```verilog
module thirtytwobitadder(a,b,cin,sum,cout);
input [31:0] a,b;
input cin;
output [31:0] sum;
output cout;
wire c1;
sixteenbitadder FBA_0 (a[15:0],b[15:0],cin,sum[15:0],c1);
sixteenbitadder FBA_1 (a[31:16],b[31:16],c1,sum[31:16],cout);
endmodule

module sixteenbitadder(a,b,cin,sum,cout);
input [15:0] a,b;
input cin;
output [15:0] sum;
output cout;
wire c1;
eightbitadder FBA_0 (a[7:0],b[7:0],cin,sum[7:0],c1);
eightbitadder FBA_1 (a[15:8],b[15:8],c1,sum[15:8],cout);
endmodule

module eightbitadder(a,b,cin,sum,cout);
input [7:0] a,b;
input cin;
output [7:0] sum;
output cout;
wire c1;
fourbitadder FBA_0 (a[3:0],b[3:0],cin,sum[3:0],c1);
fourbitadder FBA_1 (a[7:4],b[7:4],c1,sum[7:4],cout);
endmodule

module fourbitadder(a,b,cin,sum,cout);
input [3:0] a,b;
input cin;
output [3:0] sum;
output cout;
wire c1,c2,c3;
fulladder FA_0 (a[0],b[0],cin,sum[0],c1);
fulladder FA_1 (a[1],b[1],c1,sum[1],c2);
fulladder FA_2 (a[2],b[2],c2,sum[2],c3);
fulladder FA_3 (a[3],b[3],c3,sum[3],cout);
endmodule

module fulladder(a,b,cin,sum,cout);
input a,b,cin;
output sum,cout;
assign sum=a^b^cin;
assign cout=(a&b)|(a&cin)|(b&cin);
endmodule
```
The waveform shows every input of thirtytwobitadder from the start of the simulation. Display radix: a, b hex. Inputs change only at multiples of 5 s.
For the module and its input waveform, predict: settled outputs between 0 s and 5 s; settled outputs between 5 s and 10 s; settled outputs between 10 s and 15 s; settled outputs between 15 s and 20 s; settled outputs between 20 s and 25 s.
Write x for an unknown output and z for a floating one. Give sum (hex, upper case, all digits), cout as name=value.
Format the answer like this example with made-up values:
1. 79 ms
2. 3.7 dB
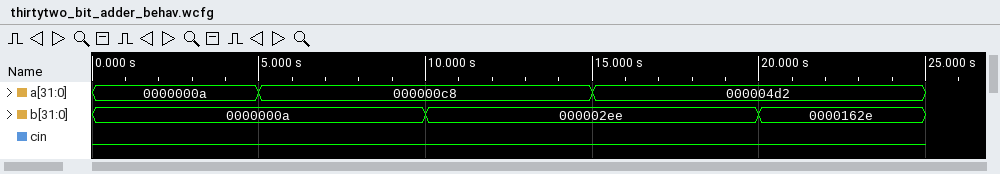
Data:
1. sum=00000014, cout=0
2. sum=000000D2, cout=0
3. sum=000003B6, cout=0
4. sum=000007C0, cout=0
5. sum=00001B00, cout=0
